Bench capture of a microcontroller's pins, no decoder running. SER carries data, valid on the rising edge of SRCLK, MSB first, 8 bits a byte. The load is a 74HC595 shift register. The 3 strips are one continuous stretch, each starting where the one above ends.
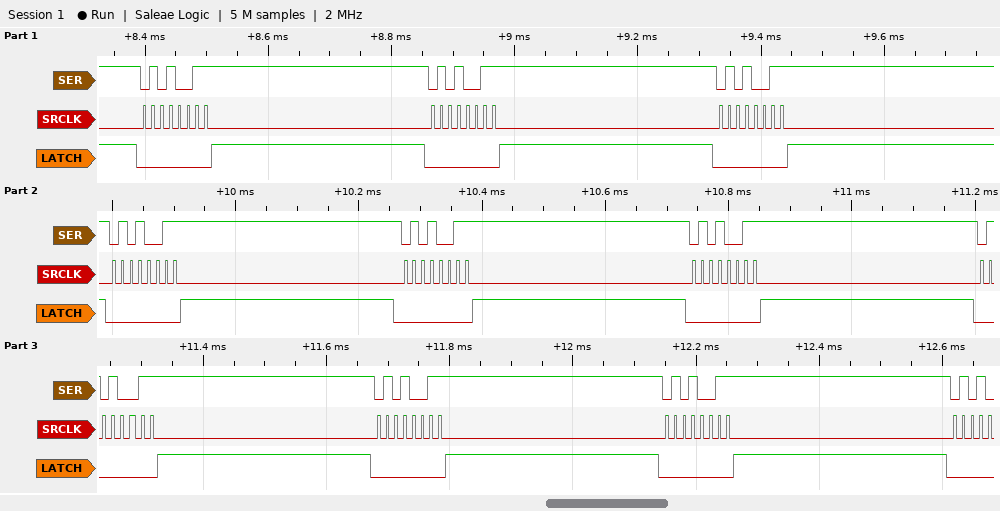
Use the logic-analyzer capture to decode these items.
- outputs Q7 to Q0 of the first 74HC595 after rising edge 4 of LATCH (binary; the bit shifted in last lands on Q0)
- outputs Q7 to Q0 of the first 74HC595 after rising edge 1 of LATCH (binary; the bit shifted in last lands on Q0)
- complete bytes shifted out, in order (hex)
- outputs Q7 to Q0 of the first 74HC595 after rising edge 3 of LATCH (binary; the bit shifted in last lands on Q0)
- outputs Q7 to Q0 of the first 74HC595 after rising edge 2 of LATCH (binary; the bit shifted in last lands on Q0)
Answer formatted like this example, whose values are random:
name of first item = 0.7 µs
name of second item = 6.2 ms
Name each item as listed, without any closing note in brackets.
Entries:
outputs Q7 to Q0 of the first 74HC595 after rising edge 4 of LATCH = 01010011
outputs Q7 to Q0 of the first 74HC595 after rising edge 1 of LATCH = 01010011
complete bytes shifted out, in order = 53 53 53 53 53 53 53 53 53
outputs Q7 to Q0 of the first 74HC595 after rising edge 3 of LATCH = 01010011
outputs Q7 to Q0 of the first 74HC595 after rising edge 2 of LATCH = 01010011
